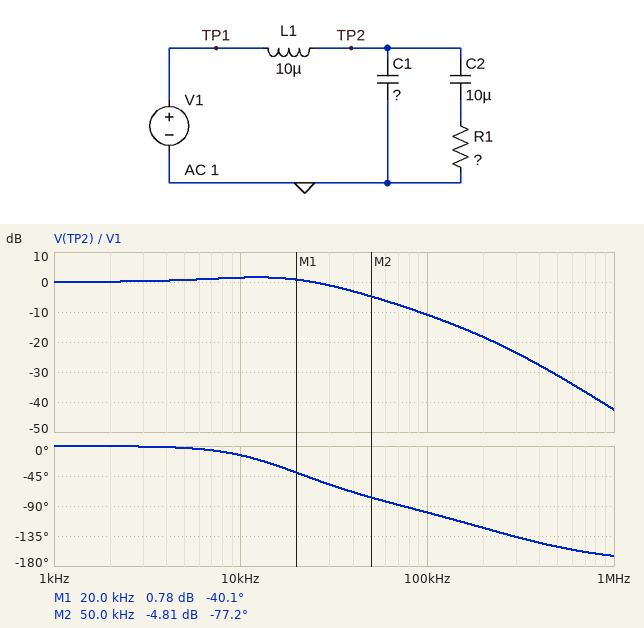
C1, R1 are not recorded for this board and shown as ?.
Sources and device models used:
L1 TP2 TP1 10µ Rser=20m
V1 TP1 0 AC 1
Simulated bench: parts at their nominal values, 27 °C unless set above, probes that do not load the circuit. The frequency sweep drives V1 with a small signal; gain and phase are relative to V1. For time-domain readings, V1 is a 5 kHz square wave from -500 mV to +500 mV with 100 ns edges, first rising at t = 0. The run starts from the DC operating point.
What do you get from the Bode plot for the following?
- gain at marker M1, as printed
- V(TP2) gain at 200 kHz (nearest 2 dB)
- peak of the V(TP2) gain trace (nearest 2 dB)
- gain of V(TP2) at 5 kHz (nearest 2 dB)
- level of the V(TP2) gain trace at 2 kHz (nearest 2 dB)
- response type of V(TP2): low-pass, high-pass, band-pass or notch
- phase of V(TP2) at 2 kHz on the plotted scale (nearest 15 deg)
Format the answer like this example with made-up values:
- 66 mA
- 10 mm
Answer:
- 0.78 dB
- -18 dB
- 2 dB
- 0 dB
- 0 dB
- low-pass
- 0 deg
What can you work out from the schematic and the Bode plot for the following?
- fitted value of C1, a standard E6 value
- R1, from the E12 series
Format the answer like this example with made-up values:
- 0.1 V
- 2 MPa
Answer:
- 330 nF
- 1.8 Ω
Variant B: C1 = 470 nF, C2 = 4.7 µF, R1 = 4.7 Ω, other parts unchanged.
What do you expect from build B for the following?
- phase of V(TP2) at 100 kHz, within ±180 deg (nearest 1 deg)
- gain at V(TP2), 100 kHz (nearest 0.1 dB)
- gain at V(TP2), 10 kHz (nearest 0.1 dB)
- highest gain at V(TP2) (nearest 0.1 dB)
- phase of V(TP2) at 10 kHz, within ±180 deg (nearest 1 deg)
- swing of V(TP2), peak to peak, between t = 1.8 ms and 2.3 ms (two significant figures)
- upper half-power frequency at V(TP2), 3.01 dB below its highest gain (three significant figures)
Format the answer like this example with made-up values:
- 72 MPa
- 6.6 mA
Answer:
- -125 deg
- -4.3 dB
- 0.7 dB
- 2.0 dB
- -6 deg
- 1.5 V
- 81.0 kHz
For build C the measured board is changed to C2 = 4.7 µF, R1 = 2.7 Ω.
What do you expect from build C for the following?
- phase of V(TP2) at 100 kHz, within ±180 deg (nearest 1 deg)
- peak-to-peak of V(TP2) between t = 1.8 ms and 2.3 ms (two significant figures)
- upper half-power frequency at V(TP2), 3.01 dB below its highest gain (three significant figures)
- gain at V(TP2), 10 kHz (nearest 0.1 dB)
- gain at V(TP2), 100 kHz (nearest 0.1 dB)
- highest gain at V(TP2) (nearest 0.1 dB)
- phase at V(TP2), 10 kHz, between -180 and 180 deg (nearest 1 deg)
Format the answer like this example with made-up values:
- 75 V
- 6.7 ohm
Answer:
- -104 deg
- 1.4 V
- 49.1 kHz
- 1.1 dB
- -7.5 dB
- 1.8 dB
- -6 deg
